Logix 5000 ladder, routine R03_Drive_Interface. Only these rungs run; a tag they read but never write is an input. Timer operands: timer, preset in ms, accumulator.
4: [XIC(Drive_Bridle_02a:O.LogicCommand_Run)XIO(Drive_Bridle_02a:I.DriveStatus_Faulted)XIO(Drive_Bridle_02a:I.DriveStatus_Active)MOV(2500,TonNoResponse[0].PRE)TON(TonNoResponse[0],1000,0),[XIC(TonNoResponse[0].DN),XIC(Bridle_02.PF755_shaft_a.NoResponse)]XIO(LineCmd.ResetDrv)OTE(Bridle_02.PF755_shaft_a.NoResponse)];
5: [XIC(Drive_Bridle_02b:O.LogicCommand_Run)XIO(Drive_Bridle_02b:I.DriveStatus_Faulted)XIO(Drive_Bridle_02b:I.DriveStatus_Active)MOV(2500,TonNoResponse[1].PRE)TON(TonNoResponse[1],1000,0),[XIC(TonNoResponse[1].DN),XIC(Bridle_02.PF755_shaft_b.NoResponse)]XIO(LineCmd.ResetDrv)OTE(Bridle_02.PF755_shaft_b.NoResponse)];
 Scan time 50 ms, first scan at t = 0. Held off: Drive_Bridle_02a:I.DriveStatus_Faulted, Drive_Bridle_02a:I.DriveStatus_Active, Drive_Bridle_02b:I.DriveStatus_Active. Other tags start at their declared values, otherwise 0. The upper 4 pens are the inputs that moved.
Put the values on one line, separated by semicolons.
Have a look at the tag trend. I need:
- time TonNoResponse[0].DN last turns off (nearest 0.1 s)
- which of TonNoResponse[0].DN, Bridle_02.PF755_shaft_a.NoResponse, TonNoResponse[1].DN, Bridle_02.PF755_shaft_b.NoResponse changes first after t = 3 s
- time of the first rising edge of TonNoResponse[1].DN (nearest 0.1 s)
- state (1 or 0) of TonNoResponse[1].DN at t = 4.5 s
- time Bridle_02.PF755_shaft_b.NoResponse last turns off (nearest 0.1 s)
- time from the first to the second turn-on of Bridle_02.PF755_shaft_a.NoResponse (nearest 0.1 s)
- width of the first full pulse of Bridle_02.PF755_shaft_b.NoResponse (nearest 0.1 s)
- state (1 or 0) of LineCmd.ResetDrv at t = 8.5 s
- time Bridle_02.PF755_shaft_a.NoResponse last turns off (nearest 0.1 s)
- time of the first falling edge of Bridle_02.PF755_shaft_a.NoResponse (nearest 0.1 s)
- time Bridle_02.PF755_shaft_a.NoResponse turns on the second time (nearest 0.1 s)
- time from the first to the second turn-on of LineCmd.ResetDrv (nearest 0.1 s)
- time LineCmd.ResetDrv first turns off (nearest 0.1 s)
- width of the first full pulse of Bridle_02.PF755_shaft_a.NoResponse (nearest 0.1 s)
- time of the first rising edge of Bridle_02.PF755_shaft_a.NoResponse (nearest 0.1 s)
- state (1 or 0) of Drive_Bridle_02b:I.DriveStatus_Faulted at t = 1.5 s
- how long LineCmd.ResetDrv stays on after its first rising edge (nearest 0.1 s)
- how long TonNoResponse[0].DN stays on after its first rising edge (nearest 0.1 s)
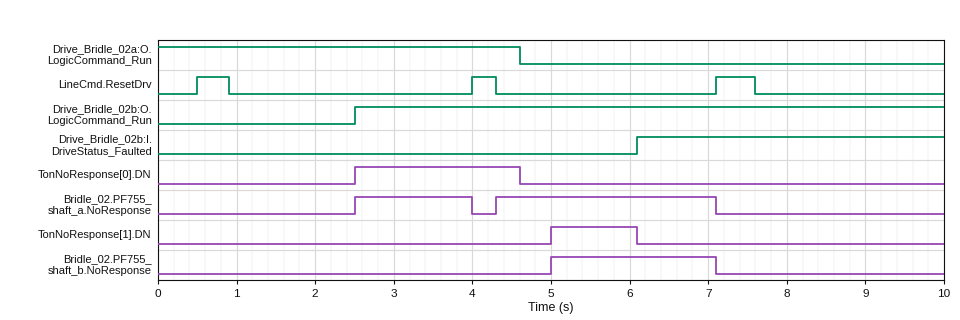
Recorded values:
4.6 s; Bridle_02.PF755_shaft_a.NoResponse; 5.0 s; 0; 7.1 s; 1.8 s; 2.1 s; 0; 7.1 s; 4.0 s; 4.3 s; 3.5 s; 0.9 s; 1.5 s; 2.5 s; 0; 0.4 s; 2.1 s
